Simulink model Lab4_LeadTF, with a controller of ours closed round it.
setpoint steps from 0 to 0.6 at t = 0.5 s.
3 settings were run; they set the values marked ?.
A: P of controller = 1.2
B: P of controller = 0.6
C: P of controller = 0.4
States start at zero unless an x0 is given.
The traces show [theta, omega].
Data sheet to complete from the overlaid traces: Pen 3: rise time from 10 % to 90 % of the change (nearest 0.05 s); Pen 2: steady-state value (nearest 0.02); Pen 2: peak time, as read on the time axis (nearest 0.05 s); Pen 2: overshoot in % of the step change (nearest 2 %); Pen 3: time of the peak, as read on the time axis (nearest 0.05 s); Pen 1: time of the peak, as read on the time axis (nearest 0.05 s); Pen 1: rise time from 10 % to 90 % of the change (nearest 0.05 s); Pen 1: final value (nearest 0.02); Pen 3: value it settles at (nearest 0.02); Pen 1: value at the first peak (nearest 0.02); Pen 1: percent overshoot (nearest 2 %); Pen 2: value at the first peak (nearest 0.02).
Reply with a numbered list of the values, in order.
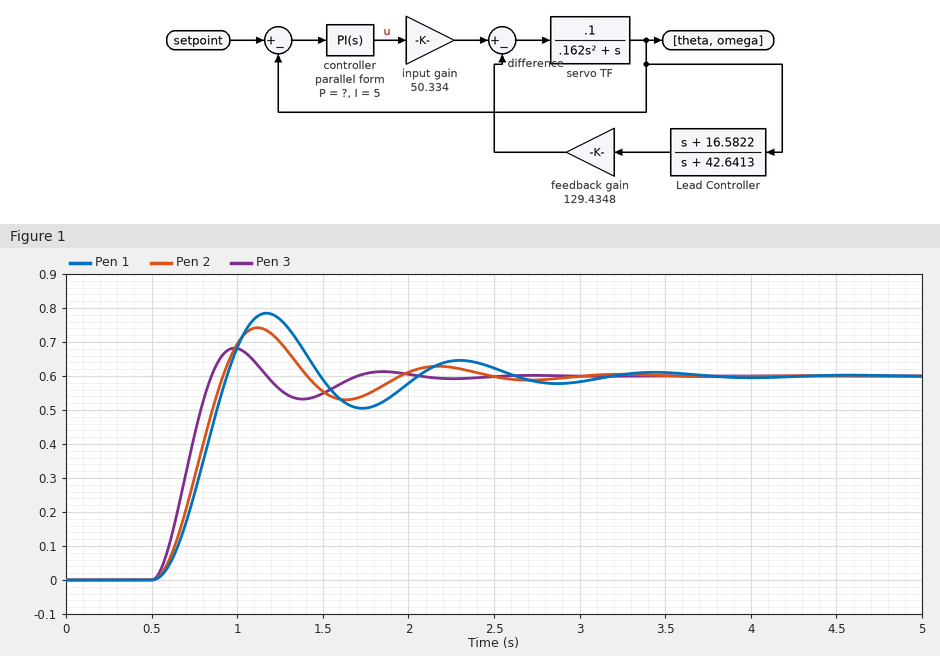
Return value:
1. 0.25 s
2. 0.60
3. 1.10 s
4. 24 %
5. 1.00 s
6. 1.15 s
7. 0.30 s
8. 0.60
9. 0.60
10. 0.78
11. 30 %
12. 0.74
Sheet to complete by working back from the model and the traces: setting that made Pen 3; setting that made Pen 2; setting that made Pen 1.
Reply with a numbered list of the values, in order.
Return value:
1. A
2. B
3. C
